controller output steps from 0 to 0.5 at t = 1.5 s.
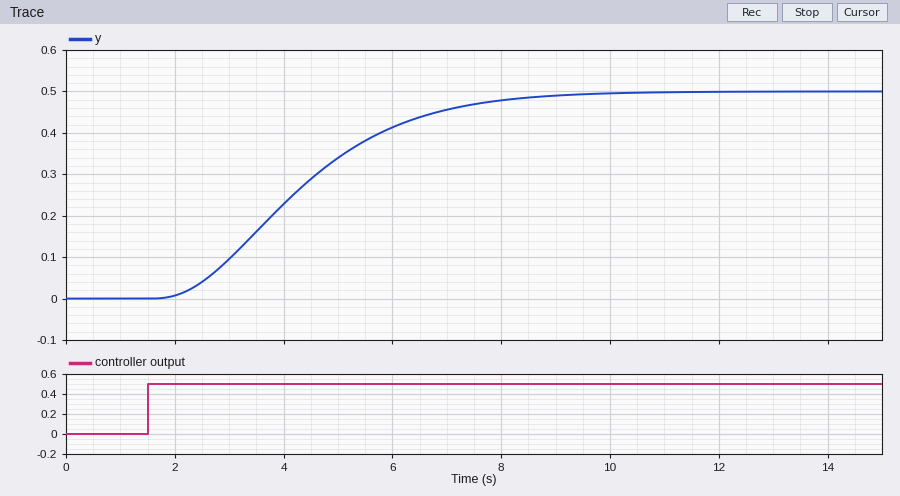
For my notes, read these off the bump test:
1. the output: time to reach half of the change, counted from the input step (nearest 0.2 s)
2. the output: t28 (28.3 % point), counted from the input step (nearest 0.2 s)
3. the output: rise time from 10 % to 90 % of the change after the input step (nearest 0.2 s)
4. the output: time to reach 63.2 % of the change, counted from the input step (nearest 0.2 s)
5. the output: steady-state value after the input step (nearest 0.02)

2.6 s
1.8 s
4.2 s
3.2 s
0.50
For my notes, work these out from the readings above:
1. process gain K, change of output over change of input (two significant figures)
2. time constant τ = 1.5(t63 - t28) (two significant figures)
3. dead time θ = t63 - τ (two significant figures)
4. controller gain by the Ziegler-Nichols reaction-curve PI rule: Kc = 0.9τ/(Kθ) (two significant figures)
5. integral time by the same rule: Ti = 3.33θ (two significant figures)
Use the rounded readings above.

1.0
2.1 s
1.1 s
1.7
3.7 s
